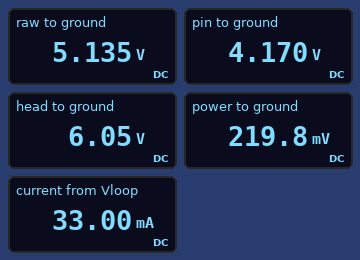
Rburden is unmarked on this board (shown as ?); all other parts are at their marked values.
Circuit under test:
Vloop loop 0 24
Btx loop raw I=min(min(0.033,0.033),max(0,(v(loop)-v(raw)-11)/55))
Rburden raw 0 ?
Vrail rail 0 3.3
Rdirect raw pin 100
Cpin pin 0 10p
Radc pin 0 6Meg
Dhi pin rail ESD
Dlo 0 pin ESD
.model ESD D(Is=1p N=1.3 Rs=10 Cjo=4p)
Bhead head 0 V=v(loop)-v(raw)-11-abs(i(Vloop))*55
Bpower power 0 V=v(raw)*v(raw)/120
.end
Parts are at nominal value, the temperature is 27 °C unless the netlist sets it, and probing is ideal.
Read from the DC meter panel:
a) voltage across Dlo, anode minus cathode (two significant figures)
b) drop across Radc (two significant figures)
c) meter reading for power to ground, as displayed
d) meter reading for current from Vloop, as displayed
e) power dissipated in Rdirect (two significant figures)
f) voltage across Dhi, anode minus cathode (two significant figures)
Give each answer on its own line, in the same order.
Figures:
-4.2 V
4.2 V
219.8 mV
33.00 mA
9.3 mW
870 mV
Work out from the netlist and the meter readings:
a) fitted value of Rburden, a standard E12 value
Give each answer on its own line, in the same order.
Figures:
220 Ω
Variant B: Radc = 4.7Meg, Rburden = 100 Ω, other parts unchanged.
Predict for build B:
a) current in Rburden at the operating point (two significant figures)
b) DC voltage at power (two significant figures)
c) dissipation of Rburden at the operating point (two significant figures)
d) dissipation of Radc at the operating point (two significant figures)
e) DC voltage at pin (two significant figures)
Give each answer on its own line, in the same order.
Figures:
33 mA
91 mV
110 mW
2.3 µW
3.3 V
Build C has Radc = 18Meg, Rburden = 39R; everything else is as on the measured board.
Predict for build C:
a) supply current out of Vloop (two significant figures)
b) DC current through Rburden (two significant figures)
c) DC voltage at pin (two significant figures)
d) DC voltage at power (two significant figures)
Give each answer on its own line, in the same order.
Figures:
33 mA
33 mA
1.3 V
14 mV
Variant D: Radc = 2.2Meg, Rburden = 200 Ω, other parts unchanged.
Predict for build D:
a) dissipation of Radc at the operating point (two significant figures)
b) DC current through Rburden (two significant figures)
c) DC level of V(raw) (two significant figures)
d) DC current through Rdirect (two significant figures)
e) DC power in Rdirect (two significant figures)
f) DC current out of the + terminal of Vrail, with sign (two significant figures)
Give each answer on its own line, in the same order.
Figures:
7.8 µW
25 mA
5.0 V
8.2 mA
6.7 mW
-8.2 mA
